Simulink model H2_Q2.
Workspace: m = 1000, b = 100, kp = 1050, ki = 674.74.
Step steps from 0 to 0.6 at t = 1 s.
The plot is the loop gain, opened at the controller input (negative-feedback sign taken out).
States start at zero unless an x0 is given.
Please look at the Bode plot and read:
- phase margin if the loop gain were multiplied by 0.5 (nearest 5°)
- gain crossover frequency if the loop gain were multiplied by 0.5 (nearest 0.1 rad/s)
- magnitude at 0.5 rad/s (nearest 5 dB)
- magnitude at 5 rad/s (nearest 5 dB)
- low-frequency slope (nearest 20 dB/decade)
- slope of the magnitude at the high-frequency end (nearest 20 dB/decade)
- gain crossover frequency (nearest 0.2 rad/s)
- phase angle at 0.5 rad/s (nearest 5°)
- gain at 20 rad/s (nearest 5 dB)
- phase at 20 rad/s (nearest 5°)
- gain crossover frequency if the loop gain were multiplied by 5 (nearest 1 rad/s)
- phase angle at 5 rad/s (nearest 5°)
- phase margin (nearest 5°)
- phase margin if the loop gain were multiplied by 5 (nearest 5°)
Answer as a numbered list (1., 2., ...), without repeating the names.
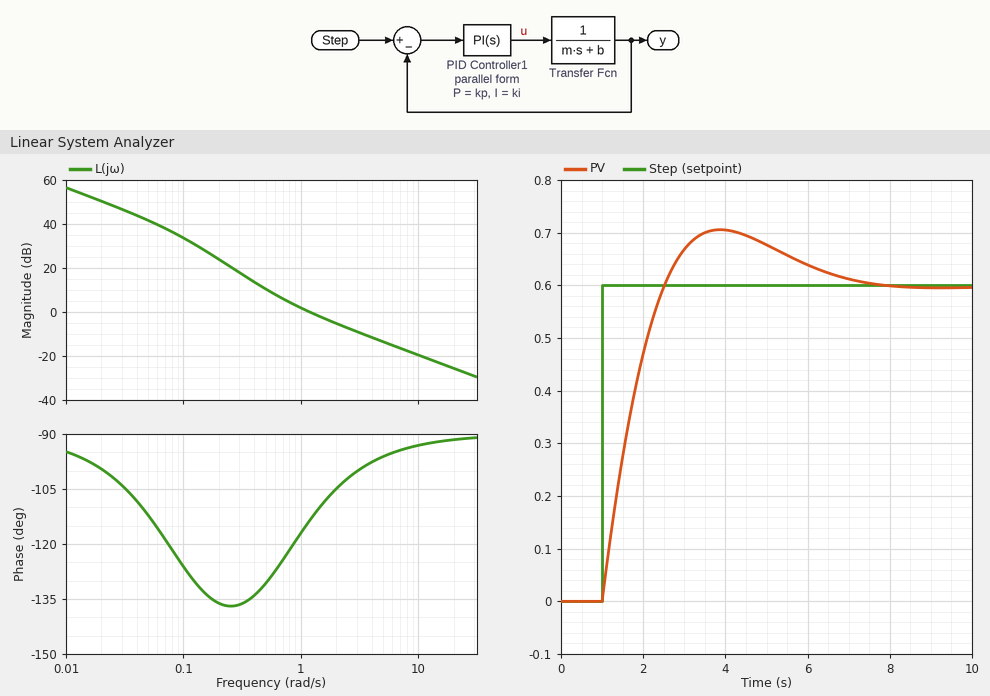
1. 55°
2. 0.7 rad/s
3. 10 dB
4. -15 dB
5. -20 dB/decade
6. -20 dB/decade
7. 1.2 rad/s
8. -130°
9. -25 dB
10. -90°
11. 5 rad/s
12. -95°
13. 65°
14. 85°
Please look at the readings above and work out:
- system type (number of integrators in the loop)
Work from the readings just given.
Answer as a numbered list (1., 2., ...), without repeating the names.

1. 1
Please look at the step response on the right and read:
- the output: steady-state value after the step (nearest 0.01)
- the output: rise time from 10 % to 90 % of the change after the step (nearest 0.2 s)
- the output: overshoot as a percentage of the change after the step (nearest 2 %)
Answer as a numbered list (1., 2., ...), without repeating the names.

1. 0.60
2. 1.2 s
3. 18 %
